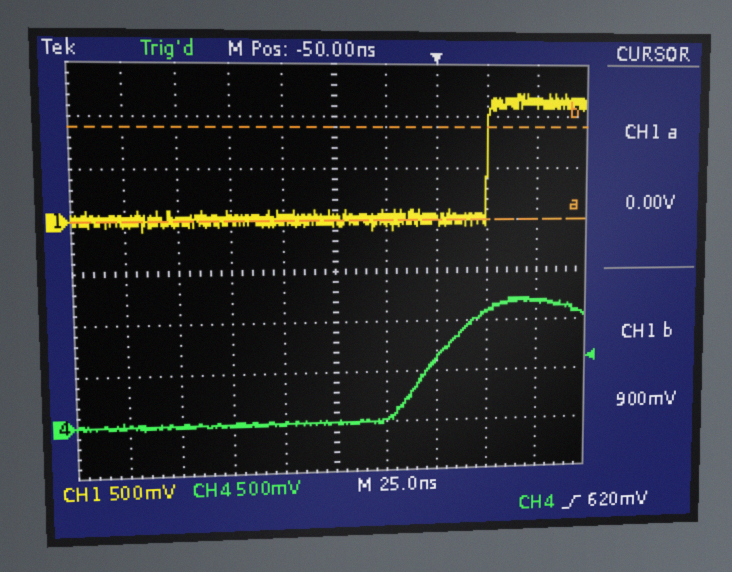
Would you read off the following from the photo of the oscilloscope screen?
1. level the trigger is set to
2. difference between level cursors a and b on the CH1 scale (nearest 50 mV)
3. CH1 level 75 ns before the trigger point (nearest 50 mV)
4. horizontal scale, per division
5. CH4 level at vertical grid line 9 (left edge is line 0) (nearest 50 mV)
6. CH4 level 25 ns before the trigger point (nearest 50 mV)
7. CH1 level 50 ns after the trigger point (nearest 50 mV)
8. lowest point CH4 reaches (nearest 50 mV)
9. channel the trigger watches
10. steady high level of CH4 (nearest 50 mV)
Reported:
620 mV
900 mV
0 mV
25 ns
1.20 V
0 mV
1.15 V
-50 mV
CH4
1.20 V
